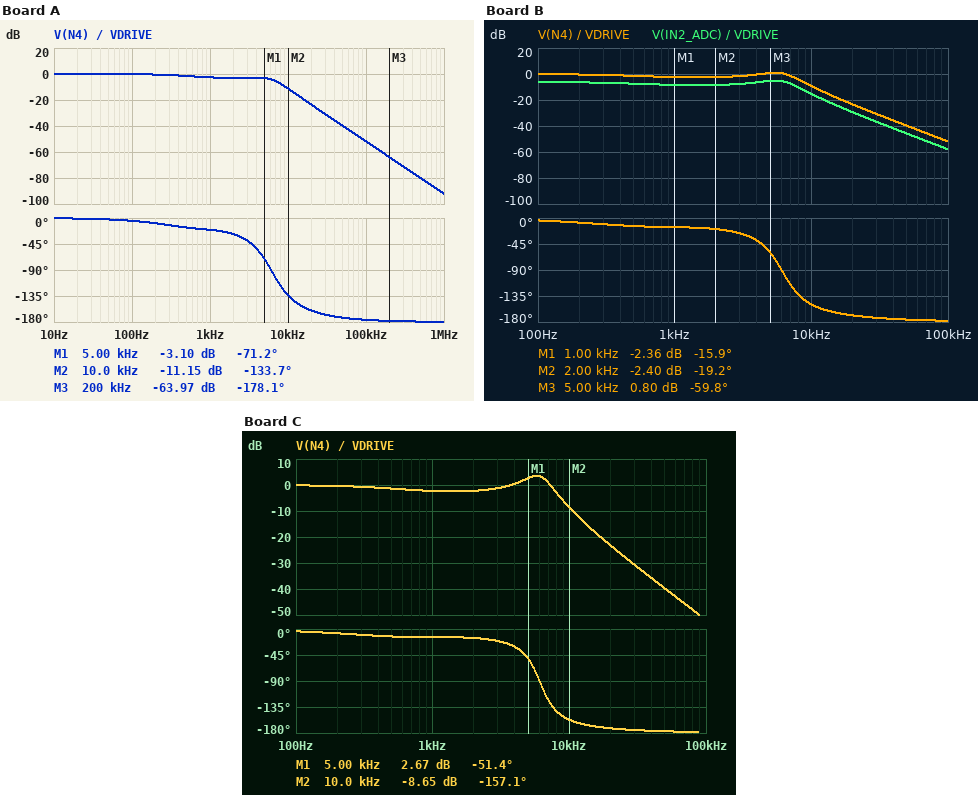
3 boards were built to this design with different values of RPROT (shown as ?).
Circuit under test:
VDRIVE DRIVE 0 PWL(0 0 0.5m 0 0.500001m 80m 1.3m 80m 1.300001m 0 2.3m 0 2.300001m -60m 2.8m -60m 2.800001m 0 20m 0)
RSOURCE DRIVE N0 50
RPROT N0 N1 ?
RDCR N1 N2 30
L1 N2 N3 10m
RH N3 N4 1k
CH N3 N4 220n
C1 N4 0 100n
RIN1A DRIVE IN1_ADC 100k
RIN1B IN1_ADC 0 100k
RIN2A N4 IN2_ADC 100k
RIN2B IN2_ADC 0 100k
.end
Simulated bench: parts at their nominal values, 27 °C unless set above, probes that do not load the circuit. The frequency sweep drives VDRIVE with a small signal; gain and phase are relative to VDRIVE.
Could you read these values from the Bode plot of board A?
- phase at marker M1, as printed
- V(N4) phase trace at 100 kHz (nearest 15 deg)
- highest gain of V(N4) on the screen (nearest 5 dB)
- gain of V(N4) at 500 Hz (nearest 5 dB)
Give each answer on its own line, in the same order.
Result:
-71.2 deg
-180 deg
0 dB
0 dB
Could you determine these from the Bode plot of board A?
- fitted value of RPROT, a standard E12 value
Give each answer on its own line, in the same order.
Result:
330 Ω
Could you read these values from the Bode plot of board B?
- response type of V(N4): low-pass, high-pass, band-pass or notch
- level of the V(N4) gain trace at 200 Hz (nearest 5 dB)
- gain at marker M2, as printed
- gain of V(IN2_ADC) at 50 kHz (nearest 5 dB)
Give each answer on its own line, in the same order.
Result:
low-pass
0 dB
-2.40 dB
-45 dB
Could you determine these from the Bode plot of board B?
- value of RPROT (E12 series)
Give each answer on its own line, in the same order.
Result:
150 Ω
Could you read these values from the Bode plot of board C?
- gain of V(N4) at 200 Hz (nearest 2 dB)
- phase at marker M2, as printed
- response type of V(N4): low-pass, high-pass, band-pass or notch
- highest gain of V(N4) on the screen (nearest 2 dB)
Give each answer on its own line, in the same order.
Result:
0 dB
-157.1 deg
low-pass
4 dB
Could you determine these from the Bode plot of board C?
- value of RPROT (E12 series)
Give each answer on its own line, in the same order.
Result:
82 Ω
